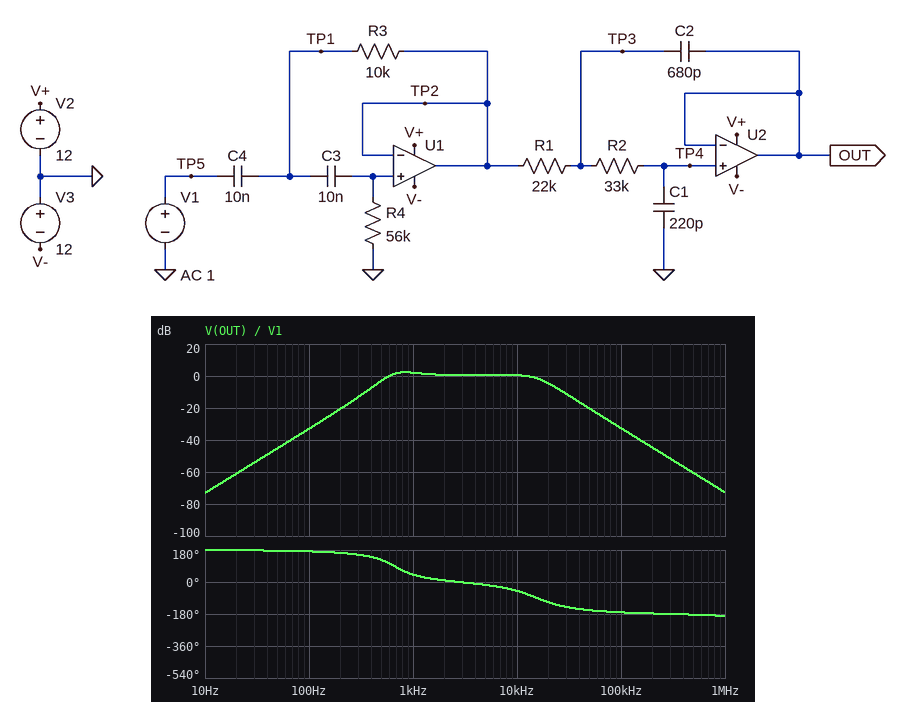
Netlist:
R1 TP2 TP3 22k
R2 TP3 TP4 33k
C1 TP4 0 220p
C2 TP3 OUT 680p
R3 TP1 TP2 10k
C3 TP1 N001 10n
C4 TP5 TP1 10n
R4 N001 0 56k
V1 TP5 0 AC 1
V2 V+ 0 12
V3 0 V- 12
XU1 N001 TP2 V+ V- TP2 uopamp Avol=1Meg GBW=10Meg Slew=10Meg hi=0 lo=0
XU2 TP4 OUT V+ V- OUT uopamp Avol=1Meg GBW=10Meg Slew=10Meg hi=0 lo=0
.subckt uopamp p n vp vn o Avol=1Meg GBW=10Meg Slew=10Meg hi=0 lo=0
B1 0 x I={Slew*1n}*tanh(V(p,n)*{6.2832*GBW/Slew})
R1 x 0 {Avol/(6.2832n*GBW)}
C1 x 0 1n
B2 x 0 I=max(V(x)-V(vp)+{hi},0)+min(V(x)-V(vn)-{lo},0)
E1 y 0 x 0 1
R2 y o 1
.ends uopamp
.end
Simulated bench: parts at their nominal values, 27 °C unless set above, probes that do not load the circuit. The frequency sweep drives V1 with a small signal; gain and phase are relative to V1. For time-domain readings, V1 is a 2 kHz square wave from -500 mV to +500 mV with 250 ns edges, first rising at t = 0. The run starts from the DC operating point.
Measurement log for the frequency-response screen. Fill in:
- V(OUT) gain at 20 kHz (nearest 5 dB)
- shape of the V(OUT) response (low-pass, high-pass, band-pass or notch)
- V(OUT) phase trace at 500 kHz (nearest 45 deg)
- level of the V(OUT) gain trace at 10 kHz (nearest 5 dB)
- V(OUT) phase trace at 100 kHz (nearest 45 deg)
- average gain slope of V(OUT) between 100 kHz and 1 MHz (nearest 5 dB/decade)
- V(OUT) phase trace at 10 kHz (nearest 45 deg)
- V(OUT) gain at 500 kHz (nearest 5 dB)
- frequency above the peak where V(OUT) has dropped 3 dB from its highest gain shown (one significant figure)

-5 dB
band-pass
-180 deg
0 dB
-180 deg
-40 dB/decade
-45 deg
-60 dB
10 kHz
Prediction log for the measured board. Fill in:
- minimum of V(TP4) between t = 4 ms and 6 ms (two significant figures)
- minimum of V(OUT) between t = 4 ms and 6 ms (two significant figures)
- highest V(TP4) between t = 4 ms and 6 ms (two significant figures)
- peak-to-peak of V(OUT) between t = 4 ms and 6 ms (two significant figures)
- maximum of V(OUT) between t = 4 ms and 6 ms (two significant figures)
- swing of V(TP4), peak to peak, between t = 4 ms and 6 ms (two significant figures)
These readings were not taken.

-820 mV
-820 mV
820 mV
1.6 V
820 mV
1.6 V
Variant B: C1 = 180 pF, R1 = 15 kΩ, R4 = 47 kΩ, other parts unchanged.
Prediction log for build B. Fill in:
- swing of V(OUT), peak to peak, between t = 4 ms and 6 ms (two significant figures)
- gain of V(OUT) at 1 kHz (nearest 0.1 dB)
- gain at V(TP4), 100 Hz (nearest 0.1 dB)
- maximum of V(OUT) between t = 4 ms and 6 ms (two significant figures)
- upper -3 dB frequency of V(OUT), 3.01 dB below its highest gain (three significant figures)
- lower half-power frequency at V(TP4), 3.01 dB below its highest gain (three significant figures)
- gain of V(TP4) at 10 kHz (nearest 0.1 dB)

1.8 V
1.7 dB
-34.5 dB
890 mV
21.3 kHz
622 Hz
0.6 dB
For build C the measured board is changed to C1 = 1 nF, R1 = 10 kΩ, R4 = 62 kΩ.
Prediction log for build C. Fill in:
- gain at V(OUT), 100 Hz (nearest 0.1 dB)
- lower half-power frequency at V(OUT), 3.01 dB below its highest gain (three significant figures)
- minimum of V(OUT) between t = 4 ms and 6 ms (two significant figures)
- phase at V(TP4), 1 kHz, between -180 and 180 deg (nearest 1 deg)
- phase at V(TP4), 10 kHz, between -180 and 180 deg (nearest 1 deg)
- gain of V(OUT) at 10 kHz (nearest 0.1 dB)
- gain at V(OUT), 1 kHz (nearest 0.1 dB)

-32.1 dB
535 Hz
-550 mV
26 deg
-85 deg
-8.6 dB
1.9 dB
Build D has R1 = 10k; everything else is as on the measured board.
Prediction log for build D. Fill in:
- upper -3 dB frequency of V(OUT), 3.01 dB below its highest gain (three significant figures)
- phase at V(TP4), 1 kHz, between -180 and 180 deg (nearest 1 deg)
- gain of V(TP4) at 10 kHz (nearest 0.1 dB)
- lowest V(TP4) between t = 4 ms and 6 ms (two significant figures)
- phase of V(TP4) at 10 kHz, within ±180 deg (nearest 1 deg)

16.4 kHz
43 deg
0 dB
-780 mV
-33 deg
